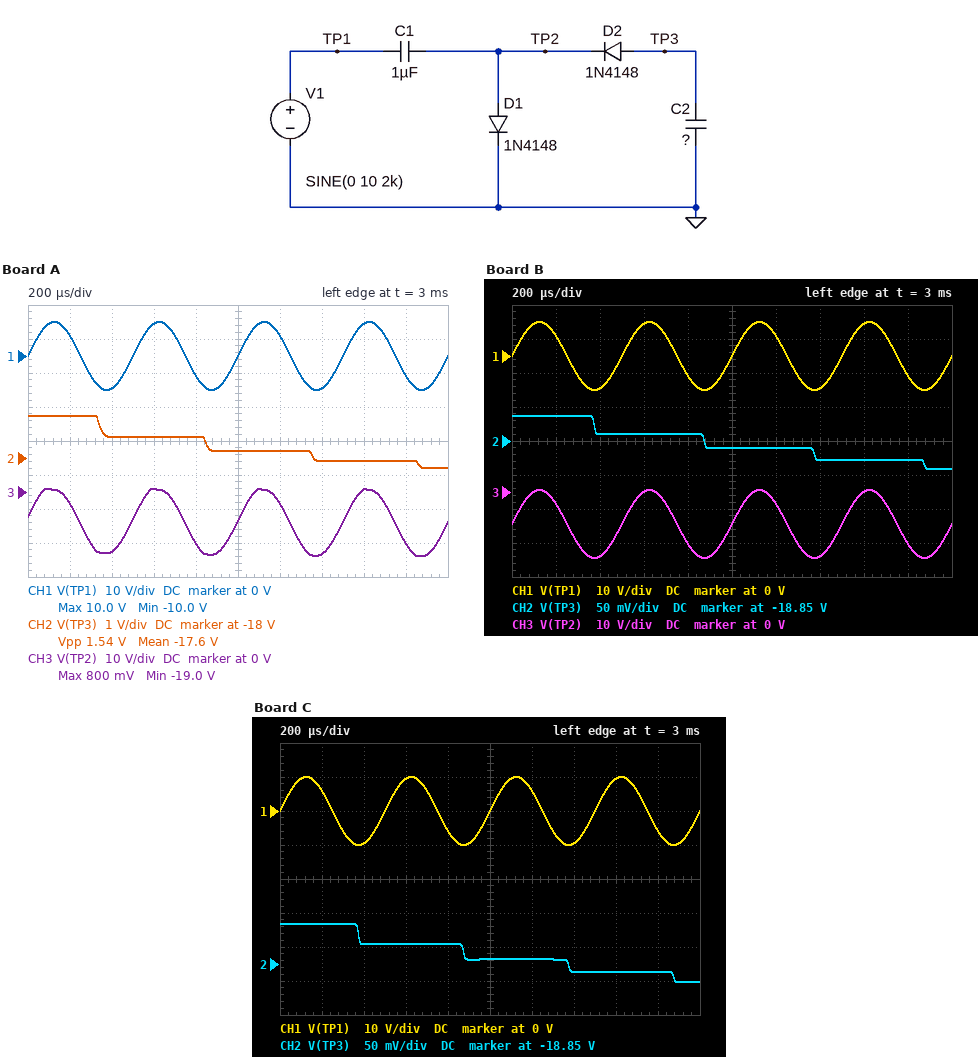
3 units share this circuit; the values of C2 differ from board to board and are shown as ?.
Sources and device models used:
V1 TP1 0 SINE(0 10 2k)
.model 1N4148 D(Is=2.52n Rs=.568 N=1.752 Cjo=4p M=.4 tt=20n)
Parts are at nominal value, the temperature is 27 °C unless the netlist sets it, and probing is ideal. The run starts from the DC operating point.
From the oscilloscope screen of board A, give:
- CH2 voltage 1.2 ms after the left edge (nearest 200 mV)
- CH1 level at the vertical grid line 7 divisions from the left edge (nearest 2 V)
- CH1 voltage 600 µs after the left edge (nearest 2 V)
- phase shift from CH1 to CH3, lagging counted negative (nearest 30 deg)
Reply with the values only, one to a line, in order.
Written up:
-17.8 V
-10 V
10 V
0 deg
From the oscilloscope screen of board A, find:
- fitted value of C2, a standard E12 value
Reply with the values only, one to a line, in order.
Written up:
2.2 µF
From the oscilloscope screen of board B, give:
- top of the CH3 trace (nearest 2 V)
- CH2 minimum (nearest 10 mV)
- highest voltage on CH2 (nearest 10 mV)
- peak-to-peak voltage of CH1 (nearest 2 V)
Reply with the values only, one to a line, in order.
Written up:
0 V
-18.89 V
-18.81 V
20 V
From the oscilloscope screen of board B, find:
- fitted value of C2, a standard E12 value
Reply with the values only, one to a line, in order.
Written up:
330 nF
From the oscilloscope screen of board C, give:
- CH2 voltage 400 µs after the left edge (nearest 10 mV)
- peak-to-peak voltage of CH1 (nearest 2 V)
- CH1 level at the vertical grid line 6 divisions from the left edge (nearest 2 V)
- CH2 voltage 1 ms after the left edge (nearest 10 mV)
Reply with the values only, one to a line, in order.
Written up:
-18.82 V
20 V
6 V
-18.84 V
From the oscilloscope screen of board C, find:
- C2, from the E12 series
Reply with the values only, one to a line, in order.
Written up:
390 nF
